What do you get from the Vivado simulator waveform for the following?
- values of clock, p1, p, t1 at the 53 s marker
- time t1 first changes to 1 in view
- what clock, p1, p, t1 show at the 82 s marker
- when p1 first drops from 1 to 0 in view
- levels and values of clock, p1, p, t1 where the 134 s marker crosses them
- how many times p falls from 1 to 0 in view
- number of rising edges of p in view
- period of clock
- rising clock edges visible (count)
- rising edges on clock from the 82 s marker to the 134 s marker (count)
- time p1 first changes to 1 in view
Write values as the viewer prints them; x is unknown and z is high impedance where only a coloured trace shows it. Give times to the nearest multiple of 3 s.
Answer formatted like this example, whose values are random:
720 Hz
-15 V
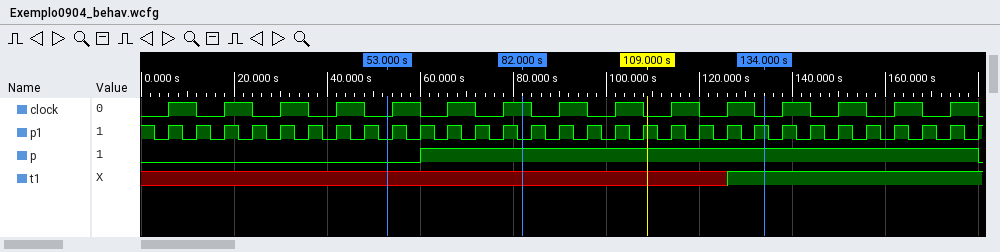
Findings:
clock=0, p1=0, p=0, t1=x
126 s
clock=1, p1=0, p=1, t1=x
3 s
clock=0, p1=1, p=1, t1=1
1
1
12 s
15
4
6 s
